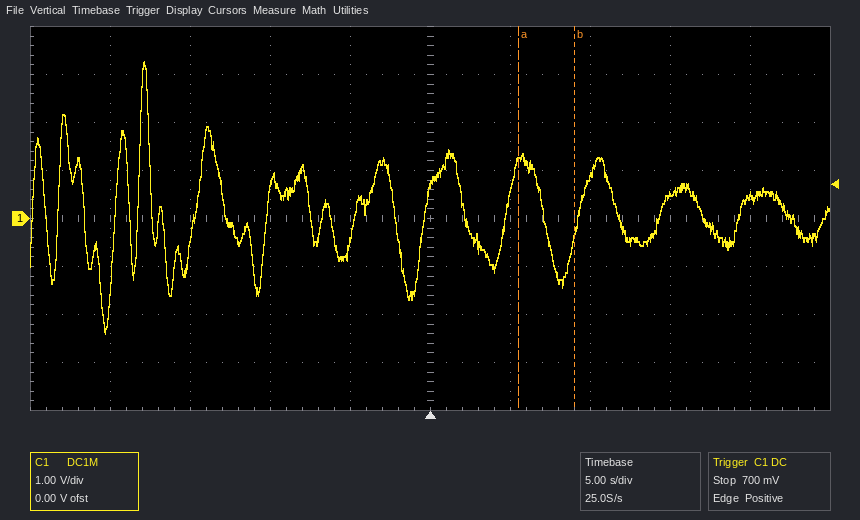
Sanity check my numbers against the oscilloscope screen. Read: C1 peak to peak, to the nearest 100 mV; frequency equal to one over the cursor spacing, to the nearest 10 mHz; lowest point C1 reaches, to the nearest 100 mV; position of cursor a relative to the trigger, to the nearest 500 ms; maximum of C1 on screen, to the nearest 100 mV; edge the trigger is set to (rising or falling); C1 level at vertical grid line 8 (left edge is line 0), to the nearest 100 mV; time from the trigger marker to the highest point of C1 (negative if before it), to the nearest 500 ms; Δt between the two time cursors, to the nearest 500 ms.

5.7 V
290 mHz
-2.4 V
+5.5 s
3.3 V
rising
500 mV
-18.0 s
3.5 s
